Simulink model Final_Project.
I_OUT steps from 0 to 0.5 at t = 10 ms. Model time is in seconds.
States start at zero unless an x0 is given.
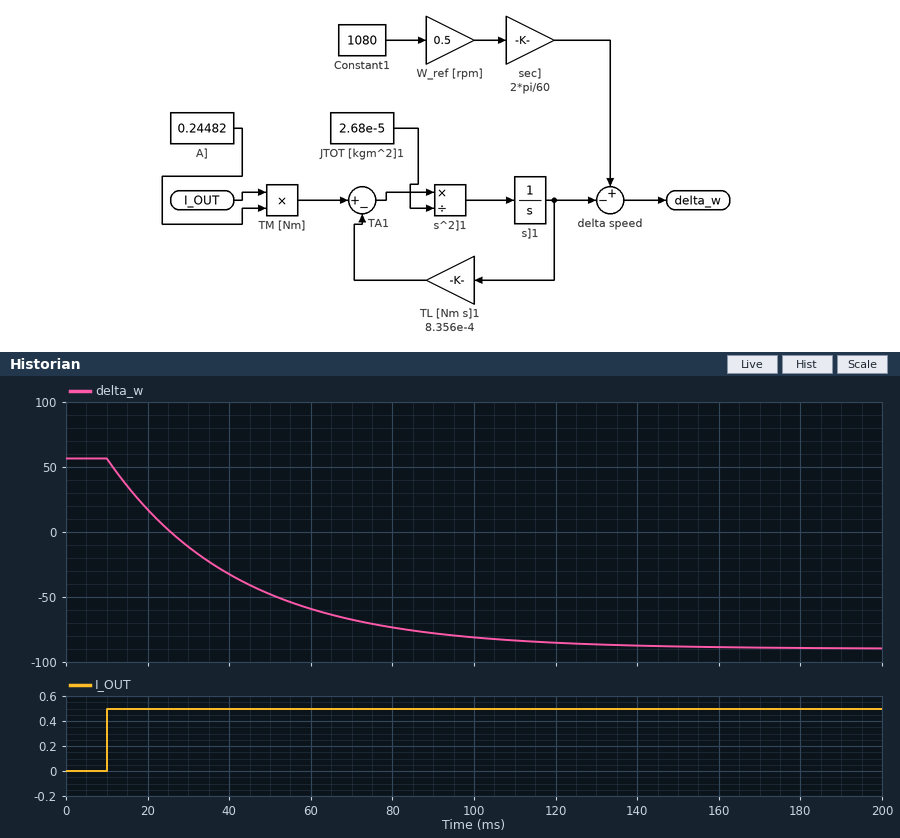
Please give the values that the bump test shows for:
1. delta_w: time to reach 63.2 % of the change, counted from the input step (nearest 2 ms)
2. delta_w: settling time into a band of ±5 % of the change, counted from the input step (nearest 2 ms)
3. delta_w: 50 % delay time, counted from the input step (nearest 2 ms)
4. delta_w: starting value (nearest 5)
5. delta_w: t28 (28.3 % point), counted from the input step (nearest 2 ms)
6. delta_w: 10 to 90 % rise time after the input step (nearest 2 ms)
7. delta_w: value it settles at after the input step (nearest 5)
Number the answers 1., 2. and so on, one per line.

1. 32 ms
2. 96 ms
3. 22 ms
4. 55
5. 10 ms
6. 70 ms
7. -90
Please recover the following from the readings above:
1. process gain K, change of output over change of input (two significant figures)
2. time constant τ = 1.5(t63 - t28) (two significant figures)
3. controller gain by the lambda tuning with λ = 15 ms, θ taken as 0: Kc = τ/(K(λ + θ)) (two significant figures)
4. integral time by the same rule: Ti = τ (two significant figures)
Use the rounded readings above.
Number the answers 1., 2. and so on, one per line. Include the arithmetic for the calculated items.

1. (-90 - 55) / 0.5 = -290
2. 1.5 × (32 - 10) = 33 ms
3. 33 / (-290 × (15 + 0)) = -0.0076
4. 33 ms
